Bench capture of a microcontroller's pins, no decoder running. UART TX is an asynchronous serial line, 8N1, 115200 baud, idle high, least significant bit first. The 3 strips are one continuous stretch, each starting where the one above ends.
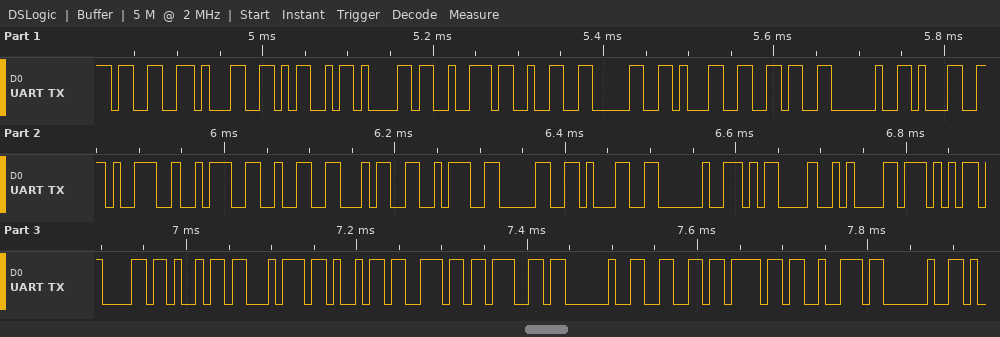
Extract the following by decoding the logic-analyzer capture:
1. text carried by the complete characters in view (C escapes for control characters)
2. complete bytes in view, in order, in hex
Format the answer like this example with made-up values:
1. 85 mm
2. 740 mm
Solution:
1. "31Mar2016 19:24:01 \r\nWaiting for "
2. 33 31 4D 61 72 32 30 31 36 20 31 39 3A 32 34 3A 30 31 20 0D 0A 57 61 69 74 69 6E 67 20 66 6F 72 20
